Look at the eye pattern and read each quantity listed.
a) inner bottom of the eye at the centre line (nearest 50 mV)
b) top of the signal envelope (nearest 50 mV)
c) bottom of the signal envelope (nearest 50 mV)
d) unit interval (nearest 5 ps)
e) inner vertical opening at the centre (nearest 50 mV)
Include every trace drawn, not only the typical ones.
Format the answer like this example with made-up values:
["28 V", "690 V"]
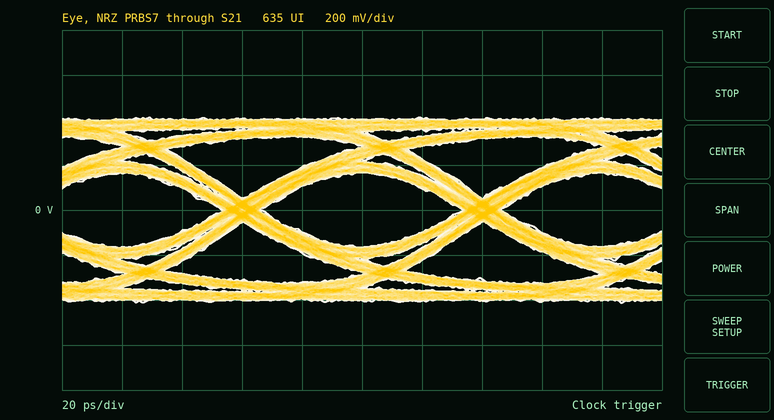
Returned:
["-150 mV", "400 mV", "-400 mV", "80 ps", "350 mV"]
